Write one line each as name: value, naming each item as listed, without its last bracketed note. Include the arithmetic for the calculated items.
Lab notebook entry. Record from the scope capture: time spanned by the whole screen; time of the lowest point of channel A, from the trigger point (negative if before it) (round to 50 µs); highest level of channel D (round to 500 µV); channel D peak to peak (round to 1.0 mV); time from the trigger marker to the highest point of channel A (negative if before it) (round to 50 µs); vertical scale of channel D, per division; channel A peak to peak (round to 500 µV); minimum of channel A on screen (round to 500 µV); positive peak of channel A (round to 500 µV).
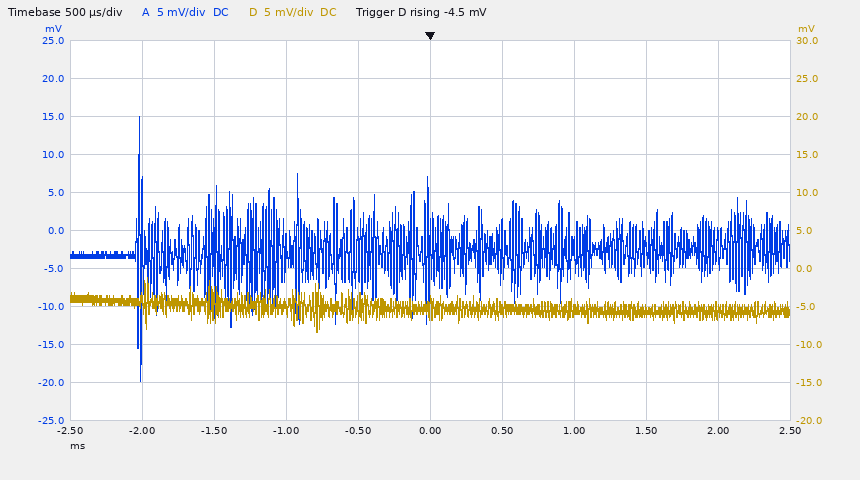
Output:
time spanned by the whole screen: 5 ms
time of the lowest point of channel A, from the trigger point (negative if before it): -2.00 ms
highest level of channel D: -1.0 mV
channel D peak to peak: 7.0 mV
time from the trigger marker to the highest point of channel A (negative if before it): -2.00 ms
vertical scale of channel D, per division: 5 mV
channel A peak to peak: 15.0 mV − (-19.5 mV) = 34.5 mV
minimum of channel A on screen: -19.5 mV
positive peak of channel A: 15.0 mV
